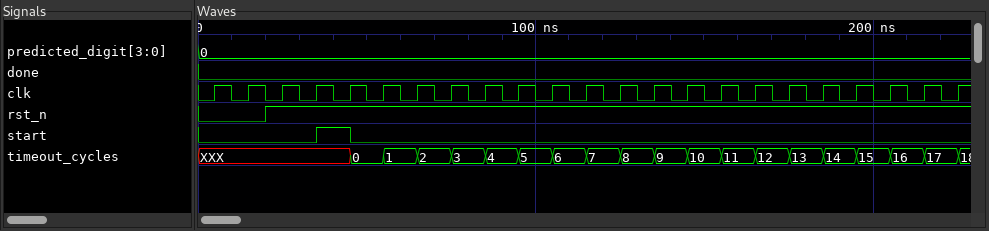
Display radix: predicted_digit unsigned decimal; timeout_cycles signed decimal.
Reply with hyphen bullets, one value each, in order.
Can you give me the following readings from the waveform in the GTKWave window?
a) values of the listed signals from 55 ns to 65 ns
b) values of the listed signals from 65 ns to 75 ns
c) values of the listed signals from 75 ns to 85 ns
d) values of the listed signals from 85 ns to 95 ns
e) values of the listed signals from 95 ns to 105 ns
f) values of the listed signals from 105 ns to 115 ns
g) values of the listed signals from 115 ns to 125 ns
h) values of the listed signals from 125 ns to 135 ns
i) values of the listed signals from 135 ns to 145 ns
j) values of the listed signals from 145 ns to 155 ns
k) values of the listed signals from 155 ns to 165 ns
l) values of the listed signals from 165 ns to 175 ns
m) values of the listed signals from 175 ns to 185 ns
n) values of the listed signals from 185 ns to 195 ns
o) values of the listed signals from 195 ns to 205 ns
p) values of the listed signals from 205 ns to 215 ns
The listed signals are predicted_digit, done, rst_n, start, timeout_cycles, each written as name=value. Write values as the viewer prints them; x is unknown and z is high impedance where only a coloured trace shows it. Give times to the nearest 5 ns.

- predicted_digit=0, done=0, rst_n=1, start=0, timeout_cycles=1
- predicted_digit=0, done=0, rst_n=1, start=0, timeout_cycles=2
- predicted_digit=0, done=0, rst_n=1, start=0, timeout_cycles=3
- predicted_digit=0, done=0, rst_n=1, start=0, timeout_cycles=4
- predicted_digit=0, done=0, rst_n=1, start=0, timeout_cycles=5
- predicted_digit=0, done=0, rst_n=1, start=0, timeout_cycles=6
- predicted_digit=0, done=0, rst_n=1, start=0, timeout_cycles=7
- predicted_digit=0, done=0, rst_n=1, start=0, timeout_cycles=8
- predicted_digit=0, done=0, rst_n=1, start=0, timeout_cycles=9
- predicted_digit=0, done=0, rst_n=1, start=0, timeout_cycles=10
- predicted_digit=0, done=0, rst_n=1, start=0, timeout_cycles=11
- predicted_digit=0, done=0, rst_n=1, start=0, timeout_cycles=12
- predicted_digit=0, done=0, rst_n=1, start=0, timeout_cycles=13
- predicted_digit=0, done=0, rst_n=1, start=0, timeout_cycles=14
- predicted_digit=0, done=0, rst_n=1, start=0, timeout_cycles=15
- predicted_digit=0, done=0, rst_n=1, start=0, timeout_cycles=16
